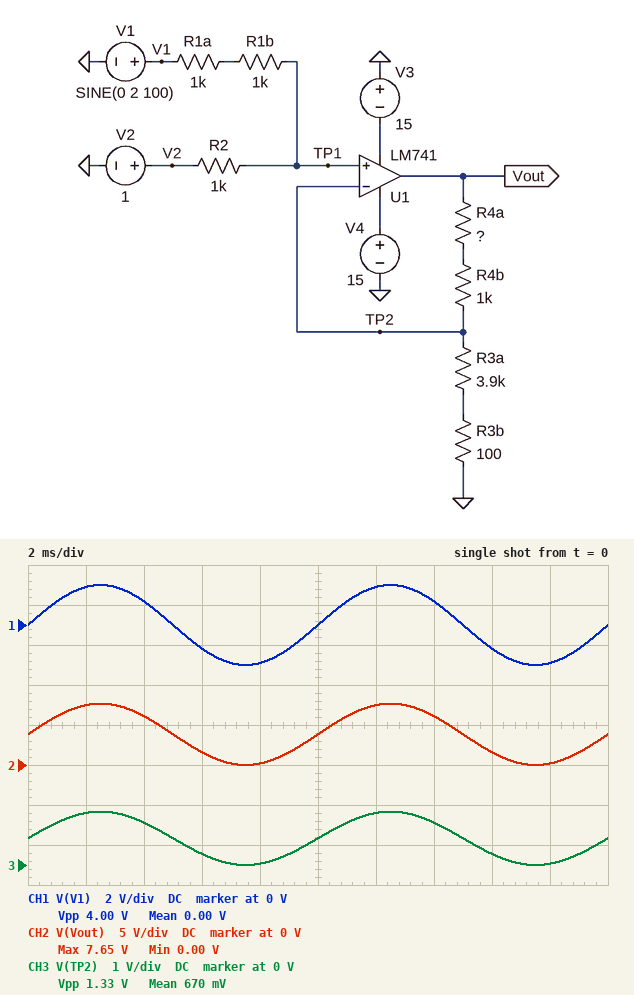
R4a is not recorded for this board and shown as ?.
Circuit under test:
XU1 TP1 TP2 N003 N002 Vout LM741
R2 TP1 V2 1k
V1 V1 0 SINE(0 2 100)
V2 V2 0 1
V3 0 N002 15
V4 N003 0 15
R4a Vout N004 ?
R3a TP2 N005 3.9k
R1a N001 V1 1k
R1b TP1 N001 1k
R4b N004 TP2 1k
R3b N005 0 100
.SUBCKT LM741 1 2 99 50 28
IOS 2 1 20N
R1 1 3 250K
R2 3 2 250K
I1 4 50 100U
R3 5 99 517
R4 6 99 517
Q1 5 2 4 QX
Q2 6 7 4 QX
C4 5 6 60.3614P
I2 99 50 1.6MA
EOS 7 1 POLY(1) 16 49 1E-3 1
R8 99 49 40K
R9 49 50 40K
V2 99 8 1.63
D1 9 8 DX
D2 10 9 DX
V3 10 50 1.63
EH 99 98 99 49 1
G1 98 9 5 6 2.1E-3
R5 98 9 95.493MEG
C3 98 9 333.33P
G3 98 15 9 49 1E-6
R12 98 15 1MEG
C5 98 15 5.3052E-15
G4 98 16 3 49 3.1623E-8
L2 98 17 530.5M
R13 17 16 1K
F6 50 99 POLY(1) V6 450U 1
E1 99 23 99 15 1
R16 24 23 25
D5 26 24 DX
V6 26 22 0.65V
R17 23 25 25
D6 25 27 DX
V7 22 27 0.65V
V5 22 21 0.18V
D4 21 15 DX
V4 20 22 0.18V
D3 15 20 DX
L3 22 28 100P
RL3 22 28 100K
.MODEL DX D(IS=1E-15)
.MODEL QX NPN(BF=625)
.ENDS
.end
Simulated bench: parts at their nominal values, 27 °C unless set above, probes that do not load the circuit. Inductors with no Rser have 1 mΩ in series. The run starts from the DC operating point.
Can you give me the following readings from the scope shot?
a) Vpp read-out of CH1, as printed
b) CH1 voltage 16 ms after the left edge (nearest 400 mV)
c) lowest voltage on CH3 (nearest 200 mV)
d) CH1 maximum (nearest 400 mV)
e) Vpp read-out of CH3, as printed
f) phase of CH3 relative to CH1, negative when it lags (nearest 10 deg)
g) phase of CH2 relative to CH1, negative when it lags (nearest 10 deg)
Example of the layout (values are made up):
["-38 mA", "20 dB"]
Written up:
["4.00 V", "-1.2 V", "0 V", "2.0 V", "1.33 V", "0 deg", "0 deg"]
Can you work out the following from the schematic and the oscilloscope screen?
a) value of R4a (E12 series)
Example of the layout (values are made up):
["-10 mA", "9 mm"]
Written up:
["18 kΩ"]
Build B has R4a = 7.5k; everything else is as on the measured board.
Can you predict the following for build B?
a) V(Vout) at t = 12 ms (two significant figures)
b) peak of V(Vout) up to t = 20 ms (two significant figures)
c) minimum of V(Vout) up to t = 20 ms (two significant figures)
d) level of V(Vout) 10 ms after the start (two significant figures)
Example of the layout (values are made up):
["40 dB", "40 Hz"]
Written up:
["4.1 V", "4.2 V", "3.9 mV", "2.1 V"]
